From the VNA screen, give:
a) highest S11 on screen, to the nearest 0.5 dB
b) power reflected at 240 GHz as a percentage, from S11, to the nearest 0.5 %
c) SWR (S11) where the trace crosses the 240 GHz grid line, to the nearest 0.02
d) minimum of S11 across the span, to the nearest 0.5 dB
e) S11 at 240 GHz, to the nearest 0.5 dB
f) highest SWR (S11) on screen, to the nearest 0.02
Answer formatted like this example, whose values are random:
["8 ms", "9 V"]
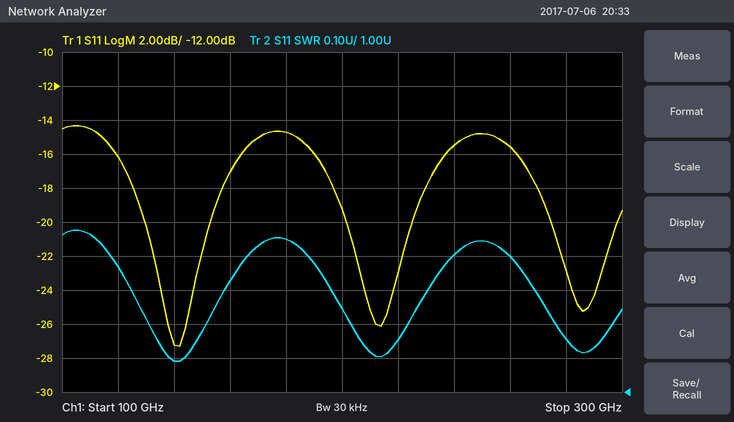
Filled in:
["-14.5 dB", "3.0 %", "1.40", "-27.5 dB", "-15.5 dB", "1.48"]
